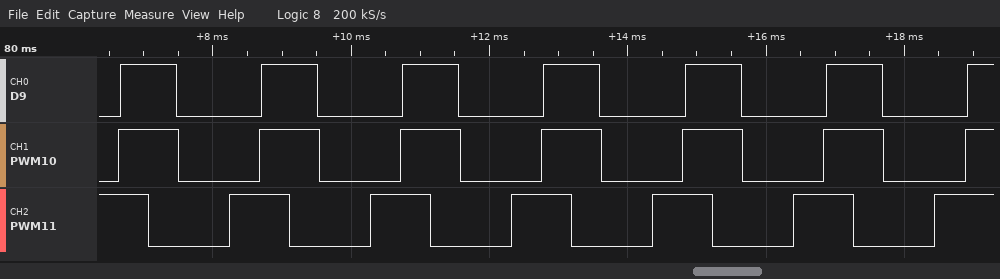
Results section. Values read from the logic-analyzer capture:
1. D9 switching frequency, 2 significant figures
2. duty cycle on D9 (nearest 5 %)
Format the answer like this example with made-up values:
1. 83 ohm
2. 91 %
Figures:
1. 490 Hz
2. 40 %
